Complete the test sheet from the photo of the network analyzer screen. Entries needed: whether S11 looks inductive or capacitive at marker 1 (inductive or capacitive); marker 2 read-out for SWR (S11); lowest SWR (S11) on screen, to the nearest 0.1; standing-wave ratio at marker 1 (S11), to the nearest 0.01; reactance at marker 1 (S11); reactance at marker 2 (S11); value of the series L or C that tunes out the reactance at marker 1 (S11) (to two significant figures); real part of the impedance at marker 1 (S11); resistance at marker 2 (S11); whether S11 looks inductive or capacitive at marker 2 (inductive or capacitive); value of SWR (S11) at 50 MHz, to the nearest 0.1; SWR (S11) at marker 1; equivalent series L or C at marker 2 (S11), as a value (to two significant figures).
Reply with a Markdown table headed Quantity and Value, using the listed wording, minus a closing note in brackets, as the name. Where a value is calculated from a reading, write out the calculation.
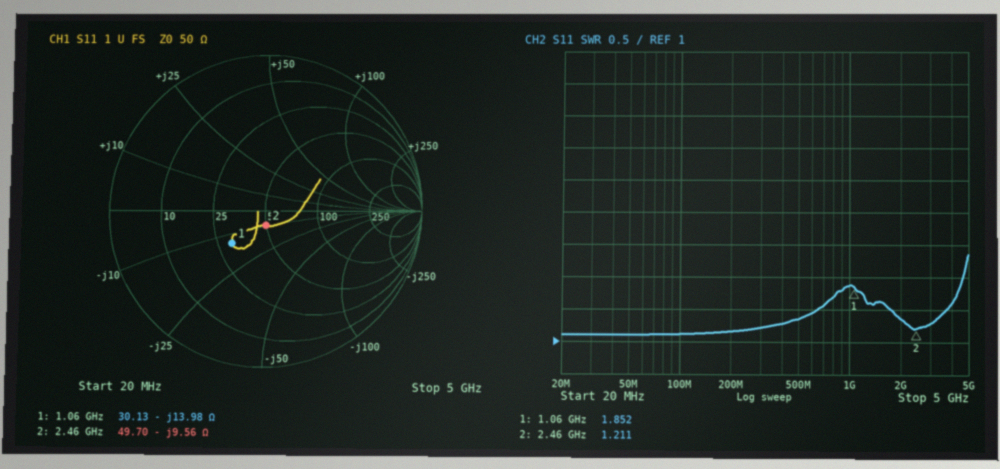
| Quantity | Value |
|---|---|
| whether S11 looks inductive or capacitive at marker 1 | capacitive |
| marker 2 read-out for SWR | 1.211 |
| lowest SWR (S11) on screen, to the nearest 0.1 | 1.1 |
| standing-wave ratio at marker 1 (S11), to the nearest 0.01 | 1.85 |
| reactance at marker 1 | -13.98 Ω |
| reactance at marker 2 | -9.56 Ω |
| value of the series L or C that tunes out the reactance at marker 1 (S11) | L = 13.98 Ω/(2π × 1.06 GHz) ≈ 2.1 nH |
| real part of the impedance at marker 1 | 30.13 Ω |
| resistance at marker 2 | 49.70 Ω |
| whether S11 looks inductive or capacitive at marker 2 | capacitive |
| value of SWR (S11) at 50 MHz, to the nearest 0.1 | 1.1 |
| SWR (S11) at marker 1 | 1.852 |
| equivalent series L or C at marker 2 (S11), as a value | C = 1/(2π × 2.46 GHz × 9.56 Ω) ≈ 6.8 pF |
